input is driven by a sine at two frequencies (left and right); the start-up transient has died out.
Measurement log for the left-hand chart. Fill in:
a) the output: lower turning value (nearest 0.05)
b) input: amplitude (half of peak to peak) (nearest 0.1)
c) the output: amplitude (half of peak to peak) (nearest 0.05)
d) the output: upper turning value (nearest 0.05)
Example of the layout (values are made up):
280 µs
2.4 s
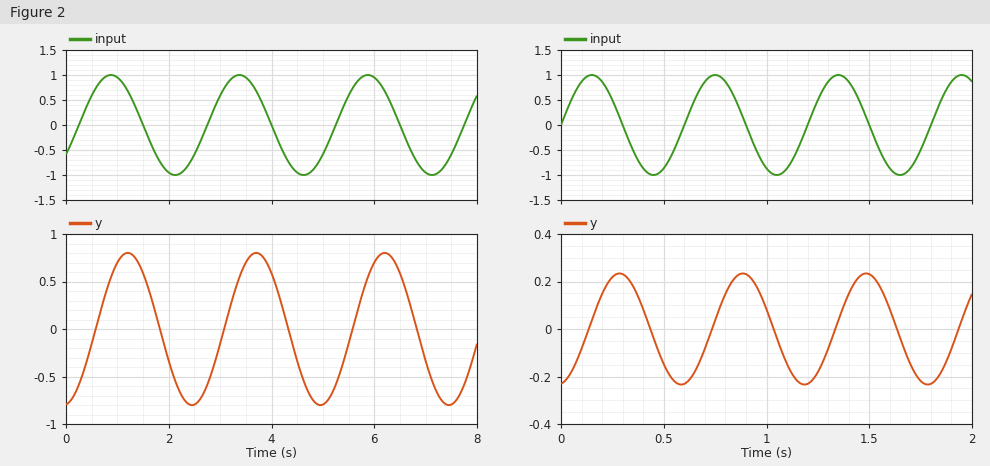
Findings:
-0.80
1.0
0.80
0.80
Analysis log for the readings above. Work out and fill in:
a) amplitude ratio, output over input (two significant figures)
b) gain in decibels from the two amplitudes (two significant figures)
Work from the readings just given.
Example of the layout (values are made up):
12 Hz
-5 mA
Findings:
0.80
-1.9 dB
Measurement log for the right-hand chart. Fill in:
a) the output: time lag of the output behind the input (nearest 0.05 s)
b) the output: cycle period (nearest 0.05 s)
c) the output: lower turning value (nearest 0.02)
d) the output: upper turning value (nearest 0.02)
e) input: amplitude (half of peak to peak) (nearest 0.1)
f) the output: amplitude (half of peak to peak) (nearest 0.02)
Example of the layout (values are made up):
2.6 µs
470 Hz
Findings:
0.15 s
0.60 s
-0.24
0.24
1.0
0.24
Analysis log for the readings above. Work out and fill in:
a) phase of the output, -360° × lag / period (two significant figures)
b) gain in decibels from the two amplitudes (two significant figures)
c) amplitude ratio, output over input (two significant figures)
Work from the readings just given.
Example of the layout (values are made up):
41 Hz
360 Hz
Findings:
-90°
-12 dB
0.24
